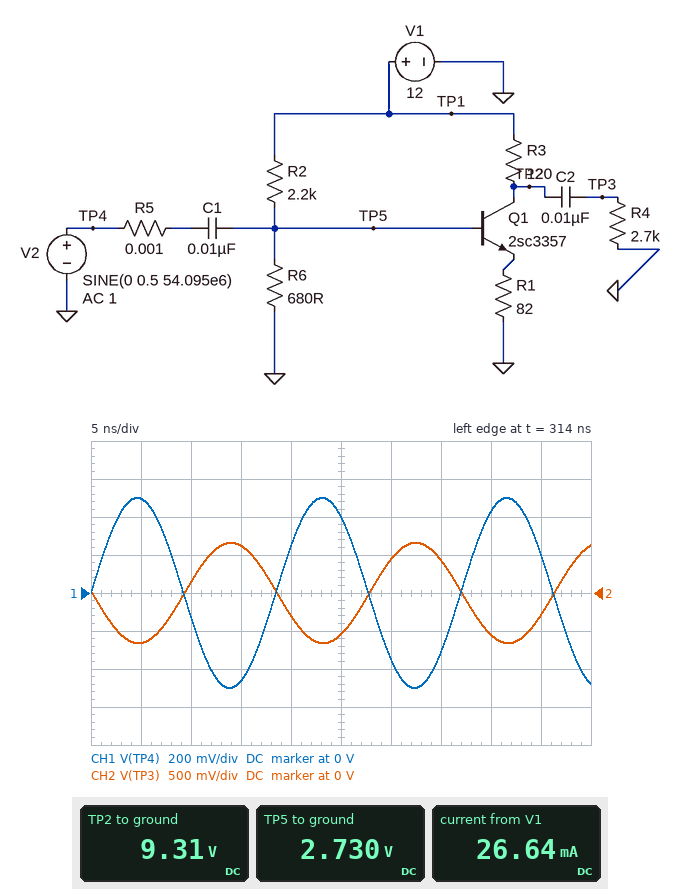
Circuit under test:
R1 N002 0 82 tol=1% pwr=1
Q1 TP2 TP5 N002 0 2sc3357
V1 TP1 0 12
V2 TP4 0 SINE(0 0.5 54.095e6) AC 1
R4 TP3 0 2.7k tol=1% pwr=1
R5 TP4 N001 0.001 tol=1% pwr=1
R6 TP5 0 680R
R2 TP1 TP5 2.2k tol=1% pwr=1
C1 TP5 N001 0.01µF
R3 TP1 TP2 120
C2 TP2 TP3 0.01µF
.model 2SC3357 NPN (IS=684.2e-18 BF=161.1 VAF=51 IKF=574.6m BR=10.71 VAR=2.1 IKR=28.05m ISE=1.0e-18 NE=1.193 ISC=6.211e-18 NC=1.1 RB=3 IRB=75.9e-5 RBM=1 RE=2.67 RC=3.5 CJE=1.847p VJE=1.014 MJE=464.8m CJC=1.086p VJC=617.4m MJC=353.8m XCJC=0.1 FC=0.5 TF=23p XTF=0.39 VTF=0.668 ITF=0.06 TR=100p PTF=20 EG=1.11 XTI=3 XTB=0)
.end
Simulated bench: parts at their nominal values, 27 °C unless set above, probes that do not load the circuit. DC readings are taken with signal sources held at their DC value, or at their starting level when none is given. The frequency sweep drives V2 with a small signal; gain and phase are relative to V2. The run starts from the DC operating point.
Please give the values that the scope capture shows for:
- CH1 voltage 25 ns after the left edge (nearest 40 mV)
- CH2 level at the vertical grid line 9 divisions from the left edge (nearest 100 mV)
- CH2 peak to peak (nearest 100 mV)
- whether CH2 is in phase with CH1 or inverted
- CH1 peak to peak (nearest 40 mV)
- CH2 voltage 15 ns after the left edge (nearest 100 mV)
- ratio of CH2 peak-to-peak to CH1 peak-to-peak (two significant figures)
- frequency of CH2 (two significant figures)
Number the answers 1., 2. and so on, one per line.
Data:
1. 400 mV
2. -300 mV
3. 1.3 V
4. inverted
5. 1.00 V
6. 600 mV
7. 1.3
8. 54 MHz
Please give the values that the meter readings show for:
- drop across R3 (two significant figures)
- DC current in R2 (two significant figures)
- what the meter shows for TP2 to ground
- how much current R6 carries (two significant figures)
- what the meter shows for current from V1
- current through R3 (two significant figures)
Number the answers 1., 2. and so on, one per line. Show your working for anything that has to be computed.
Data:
1. 12 V - 9.31 V = 2.7 V
2. (12 V - 2.73 V) / 2.2 kΩ = 4.2 mA
3. 9.31 V
4. (2.73 V) / 680 Ω = 4.0 mA
5. 26.64 mA
6. (12 V - 9.31 V) / 120 Ω = 22 mA
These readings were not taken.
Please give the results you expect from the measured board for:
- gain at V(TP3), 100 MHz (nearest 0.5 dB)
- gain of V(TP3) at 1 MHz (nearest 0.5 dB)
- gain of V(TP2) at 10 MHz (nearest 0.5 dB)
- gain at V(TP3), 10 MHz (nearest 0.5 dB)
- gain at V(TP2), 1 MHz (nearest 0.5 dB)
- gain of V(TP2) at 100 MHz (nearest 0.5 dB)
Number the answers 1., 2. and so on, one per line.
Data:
1. 2.5 dB
2. 2.5 dB
3. 2.5 dB
4. 2.5 dB
5. 2.5 dB
6. 2.5 dB
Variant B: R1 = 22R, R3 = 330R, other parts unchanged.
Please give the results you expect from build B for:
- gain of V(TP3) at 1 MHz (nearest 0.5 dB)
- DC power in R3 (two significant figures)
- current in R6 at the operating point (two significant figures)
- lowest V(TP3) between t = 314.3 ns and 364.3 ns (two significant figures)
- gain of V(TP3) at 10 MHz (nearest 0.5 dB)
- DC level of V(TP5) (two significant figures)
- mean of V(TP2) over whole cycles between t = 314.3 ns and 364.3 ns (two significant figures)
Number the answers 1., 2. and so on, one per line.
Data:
1. -8.0 dB
2. 360 mW
3. 2.5 mA
4. -170 mV
5. -7.0 dB
6. 1.7 V
7. 3.2 V
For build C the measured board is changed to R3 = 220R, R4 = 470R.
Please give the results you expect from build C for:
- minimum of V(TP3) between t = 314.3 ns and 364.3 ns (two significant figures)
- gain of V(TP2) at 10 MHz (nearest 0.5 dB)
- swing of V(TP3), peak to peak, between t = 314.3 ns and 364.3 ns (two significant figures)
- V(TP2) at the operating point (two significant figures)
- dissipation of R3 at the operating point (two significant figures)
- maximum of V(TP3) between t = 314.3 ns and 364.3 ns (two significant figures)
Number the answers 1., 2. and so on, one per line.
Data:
1. -860 mV
2. 4.5 dB
3. 1.7 V
4. 7.1 V
5. 110 mW
6. 860 mV
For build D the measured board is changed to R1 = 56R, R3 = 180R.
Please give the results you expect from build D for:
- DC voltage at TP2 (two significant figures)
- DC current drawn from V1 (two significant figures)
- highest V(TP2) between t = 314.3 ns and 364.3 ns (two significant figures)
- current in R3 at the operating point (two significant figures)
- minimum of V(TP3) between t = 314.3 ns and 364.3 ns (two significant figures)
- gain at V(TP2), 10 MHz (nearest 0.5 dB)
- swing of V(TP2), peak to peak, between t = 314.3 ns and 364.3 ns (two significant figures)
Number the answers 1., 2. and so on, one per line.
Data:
1. 6.4 V
2. 35 mA
3. 7.8 V
4. 31 mA
5. -1.4 V
6. 9.0 dB
7. 2.8 V
